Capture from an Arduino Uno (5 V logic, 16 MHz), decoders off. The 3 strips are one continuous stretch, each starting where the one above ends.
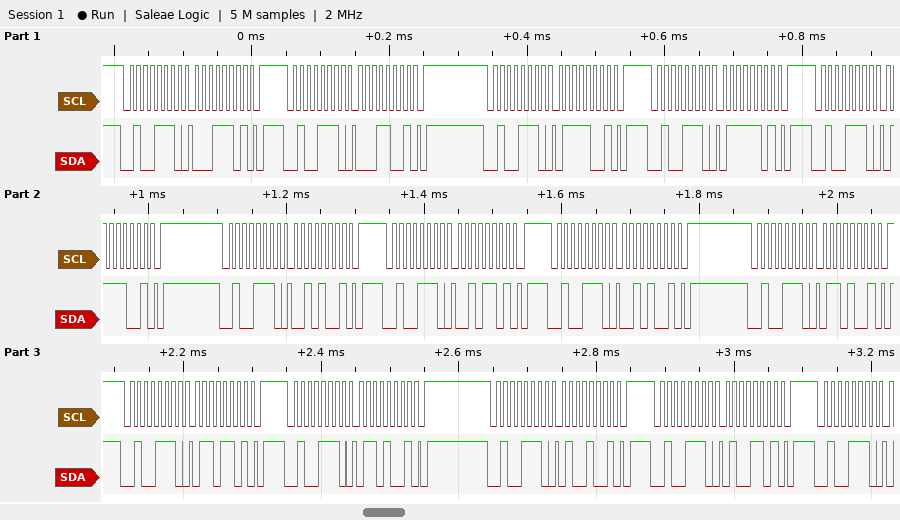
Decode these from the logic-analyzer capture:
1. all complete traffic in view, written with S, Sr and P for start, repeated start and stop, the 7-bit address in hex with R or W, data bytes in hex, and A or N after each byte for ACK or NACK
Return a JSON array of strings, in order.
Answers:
["S 27W A 1D A P S 27W A 19 A P S 27W A 79 A P S 27W A 7D A P S 27W A 79 A P S 27W A 29 A P S 27W A 2D A P S 27W A 29 A P S 27W A 69 A P S 27W A 6D A P S 27W A 69 A P S 27W A 49 A P S 27W A 4D A P S 27W A"]
